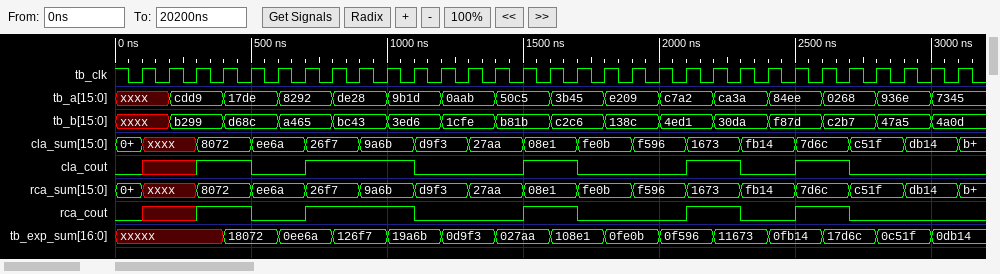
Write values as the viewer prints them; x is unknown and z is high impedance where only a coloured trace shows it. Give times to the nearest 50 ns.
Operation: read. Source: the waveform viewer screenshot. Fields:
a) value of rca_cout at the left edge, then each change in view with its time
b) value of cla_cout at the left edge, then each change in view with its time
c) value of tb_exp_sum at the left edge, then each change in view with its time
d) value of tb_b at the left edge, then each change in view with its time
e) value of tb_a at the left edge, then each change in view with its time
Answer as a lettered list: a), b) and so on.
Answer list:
a) 0, x at 100 ns, 1 at 300 ns, 0 at 500 ns, 1 at 700 ns, 0 at 1100 ns, 1 at 1500 ns, 0 at 1700 ns, 1 at 2100 ns, 0 at 2300 ns, 1 at 2500 ns, 0 at 2700 ns
b) 0, x at 100 ns, 1 at 300 ns, 0 at 500 ns, 1 at 700 ns, 0 at 1100 ns, 1 at 1500 ns, 0 at 1700 ns, 1 at 2100 ns, 0 at 2300 ns, 1 at 2500 ns, 0 at 2700 ns
c) xxxxx, 18072 at 400 ns, 0ee6a at 600 ns, 126f7 at 800 ns, 19a6b at 1000 ns, 0d9f3 at 1200 ns, 027aa at 1400 ns, 108e1 at 1600 ns, 0fe0b at 1800 ns, 0f596 at 2000 ns, 11673 at 2200 ns, 0fb14 at 2400 ns, 17d6c at 2600 ns, 0c51f at 2800 ns, 0db14 at 3000 ns
d) xxxx, b299 at 200 ns, d68c at 400 ns, a465 at 600 ns, bc43 at 800 ns, 3ed6 at 1000 ns, 1cfe at 1200 ns, b81b at 1400 ns, c2c6 at 1600 ns, 138c at 1800 ns, 4ed1 at 2000 ns, 30da at 2200 ns, f87d at 2400 ns, c2b7 at 2600 ns, 47a5 at 2800 ns, 4a0d at 3000 ns
e) xxxx, cdd9 at 200 ns, 17de at 400 ns, 8292 at 600 ns, de28 at 800 ns, 9b1d at 1000 ns, 0aab at 1200 ns, 50c5 at 1400 ns, 3b45 at 1600 ns, e209 at 1800 ns, c7a2 at 2000 ns, ca3a at 2200 ns, 84ee at 2400 ns, 0268 at 2600 ns, 936e at 2800 ns, 7345 at 3000 ns
